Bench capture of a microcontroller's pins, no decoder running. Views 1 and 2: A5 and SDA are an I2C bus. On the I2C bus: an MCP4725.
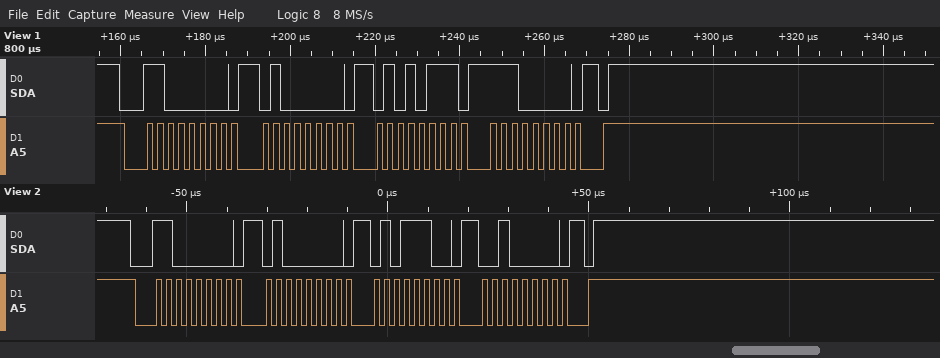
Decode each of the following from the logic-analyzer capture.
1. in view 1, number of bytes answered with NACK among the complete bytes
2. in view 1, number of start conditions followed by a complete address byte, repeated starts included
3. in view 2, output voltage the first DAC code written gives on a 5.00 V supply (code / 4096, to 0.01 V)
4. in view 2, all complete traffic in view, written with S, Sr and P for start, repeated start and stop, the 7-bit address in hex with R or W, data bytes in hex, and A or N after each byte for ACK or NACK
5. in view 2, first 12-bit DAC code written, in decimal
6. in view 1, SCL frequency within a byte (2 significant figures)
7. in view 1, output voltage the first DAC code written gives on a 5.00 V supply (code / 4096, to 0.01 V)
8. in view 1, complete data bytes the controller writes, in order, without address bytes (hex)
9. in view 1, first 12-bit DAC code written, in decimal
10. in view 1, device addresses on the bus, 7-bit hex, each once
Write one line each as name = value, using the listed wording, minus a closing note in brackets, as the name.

in view 1, number of bytes answered with NACK among the complete bytes = 0
in view 1, number of start conditions followed by a complete address byte, repeated starts included = 1
in view 2, output voltage the first DAC code written gives on a 5.00 V supply = 1.80 V
in view 2, all complete traffic in view, written with S, Sr and P for start, repeated start and stop, the 7-bit address in hex with R or W, data bytes in hex, and A or N after each byte for ACK or NACK = S 60W A 40 A 5C A 20 A P
in view 2, first 12-bit DAC code written, in decimal = 1474
in view 1, SCL frequency within a byte = 400 kHz
in view 1, output voltage the first DAC code written gives on a 5.00 V supply = 1.72 V
in view 1, complete data bytes the controller writes, in order, without address bytes = 40 57 E0
in view 1, first 12-bit DAC code written, in decimal = 1406
in view 1, device addresses on the bus, 7-bit hex, each once = 0x60
